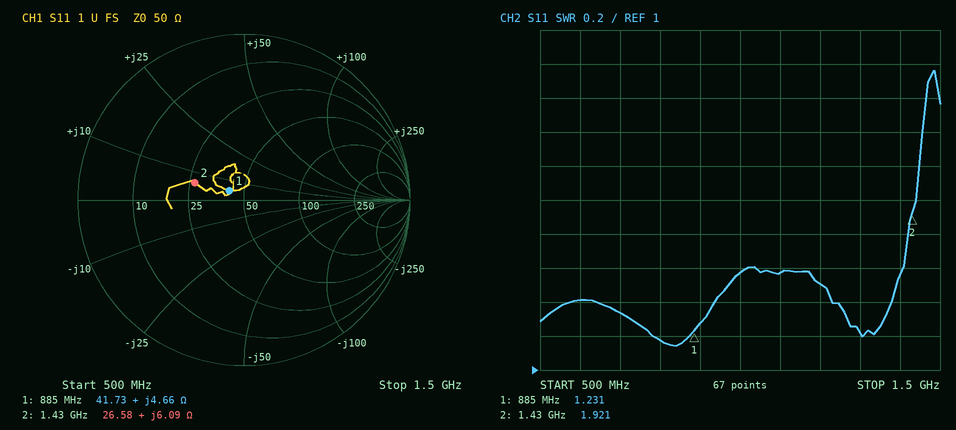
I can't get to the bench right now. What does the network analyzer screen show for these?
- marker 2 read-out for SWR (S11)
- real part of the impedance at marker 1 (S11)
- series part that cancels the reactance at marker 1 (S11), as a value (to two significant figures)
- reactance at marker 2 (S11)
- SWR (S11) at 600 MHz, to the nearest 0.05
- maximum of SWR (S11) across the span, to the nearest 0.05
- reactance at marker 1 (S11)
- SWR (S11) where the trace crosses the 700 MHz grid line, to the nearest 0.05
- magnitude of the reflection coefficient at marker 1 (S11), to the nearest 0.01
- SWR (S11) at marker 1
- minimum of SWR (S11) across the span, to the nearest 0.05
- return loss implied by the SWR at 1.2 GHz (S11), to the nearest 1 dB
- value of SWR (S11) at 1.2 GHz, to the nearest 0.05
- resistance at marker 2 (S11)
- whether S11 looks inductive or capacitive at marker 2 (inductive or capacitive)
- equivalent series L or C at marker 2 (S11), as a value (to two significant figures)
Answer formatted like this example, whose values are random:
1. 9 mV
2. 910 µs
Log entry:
1. 1.921
2. 41.73 Ω
3. 39 pF
4. +6.09 Ω
5. 1.40
6. 2.75
7. +4.66 Ω
8. 1.35
9. 0.10
10. 1.231
11. 1.15
12. 14 dB
13. 1.50
14. 26.58 Ω
15. inductive
16. 680 pH
